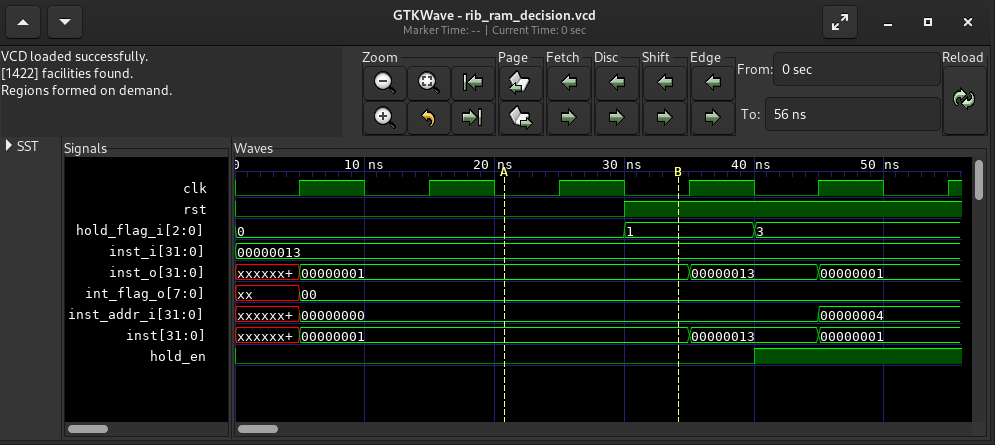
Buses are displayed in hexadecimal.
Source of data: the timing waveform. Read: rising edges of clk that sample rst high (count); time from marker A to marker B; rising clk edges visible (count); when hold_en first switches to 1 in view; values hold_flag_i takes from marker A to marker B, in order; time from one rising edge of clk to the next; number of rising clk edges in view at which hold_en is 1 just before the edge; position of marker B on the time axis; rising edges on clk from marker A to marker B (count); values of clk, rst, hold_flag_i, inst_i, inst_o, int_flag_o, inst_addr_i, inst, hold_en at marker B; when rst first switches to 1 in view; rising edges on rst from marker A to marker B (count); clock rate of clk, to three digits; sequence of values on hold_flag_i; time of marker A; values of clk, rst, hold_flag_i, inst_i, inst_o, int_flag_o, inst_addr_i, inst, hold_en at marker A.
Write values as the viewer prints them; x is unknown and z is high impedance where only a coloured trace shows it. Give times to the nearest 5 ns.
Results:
3
15 ns
6
40 ns
0, 1
10 ns
2
35 ns
1
clk=0, rst=1, hold_flag_i=1, inst_i=00000013, inst_o=00000001, int_flag_o=00, inst_addr_i=00000000, inst=00000001, hold_en=0
30 ns
1
100 MHz
0, 1, 3
20 ns
clk=0, rst=0, hold_flag_i=0, inst_i=00000013, inst_o=00000001, int_flag_o=00, inst_addr_i=00000000, inst=00000001, hold_en=0
